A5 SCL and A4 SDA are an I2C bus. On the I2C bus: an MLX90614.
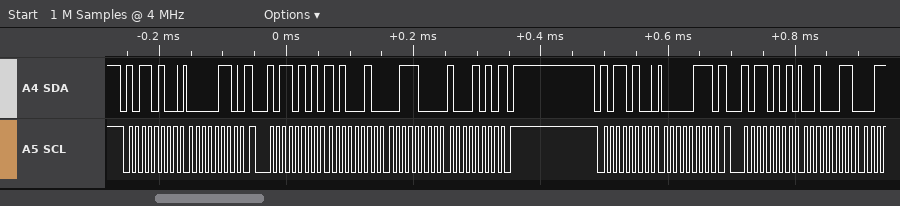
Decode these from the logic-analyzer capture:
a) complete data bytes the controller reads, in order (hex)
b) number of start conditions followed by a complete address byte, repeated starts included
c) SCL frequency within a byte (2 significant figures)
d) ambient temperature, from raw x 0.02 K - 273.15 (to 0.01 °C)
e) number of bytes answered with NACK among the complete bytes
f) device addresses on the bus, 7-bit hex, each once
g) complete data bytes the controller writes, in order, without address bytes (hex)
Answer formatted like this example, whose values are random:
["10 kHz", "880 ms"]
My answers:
["A2 38 8A 23", "4", "100 kHz", "16.81 °C", "1", "0x5A", "06 07"]
